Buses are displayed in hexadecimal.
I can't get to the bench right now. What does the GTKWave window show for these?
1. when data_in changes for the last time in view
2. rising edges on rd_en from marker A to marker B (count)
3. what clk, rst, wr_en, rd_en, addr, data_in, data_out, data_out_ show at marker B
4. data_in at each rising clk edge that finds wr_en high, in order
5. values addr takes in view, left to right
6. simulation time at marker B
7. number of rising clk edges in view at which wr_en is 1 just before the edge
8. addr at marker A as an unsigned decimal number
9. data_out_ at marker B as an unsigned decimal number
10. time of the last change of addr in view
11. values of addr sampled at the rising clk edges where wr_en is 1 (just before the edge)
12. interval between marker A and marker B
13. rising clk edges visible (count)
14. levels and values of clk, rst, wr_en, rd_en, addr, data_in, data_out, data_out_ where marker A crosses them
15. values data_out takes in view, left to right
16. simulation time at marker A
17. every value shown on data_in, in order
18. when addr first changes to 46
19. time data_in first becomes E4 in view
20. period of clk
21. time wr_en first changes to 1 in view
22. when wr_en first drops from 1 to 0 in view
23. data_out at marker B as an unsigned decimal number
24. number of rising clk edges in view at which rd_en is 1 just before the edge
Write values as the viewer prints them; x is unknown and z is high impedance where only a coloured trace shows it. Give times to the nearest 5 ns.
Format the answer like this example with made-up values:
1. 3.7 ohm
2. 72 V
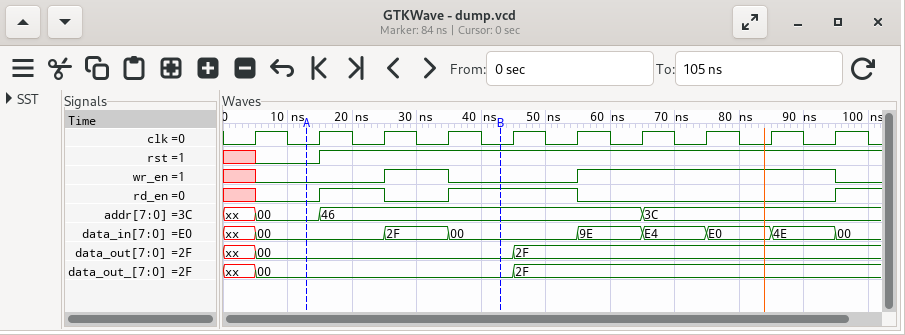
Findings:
1. 95 ns
2. 2
3. clk=0, rst=1, wr_en=0, rd_en=1, addr=46, data_in=00, data_out=00, data_out_=00
4. 2F, 9E, E4, E0, 4E
5. xx, 00, 46, 3C
6. 45 ns
7. 5
8. 0
9. 0
10. 65 ns
11. 46, 46, 3C, 3C, 3C
12. 30 ns
13. 10
14. clk=0, rst=0, wr_en=0, rd_en=0, addr=00, data_in=00, data_out=00, data_out_=00
15. xx, 00, 2F
16. 15 ns
17. xx, 00, 2F, 00, 9E, E4, E0, 4E, 00
18. 15 ns
19. 65 ns
20. 10 ns
21. 25 ns
22. 35 ns
23. 0
24. 3
